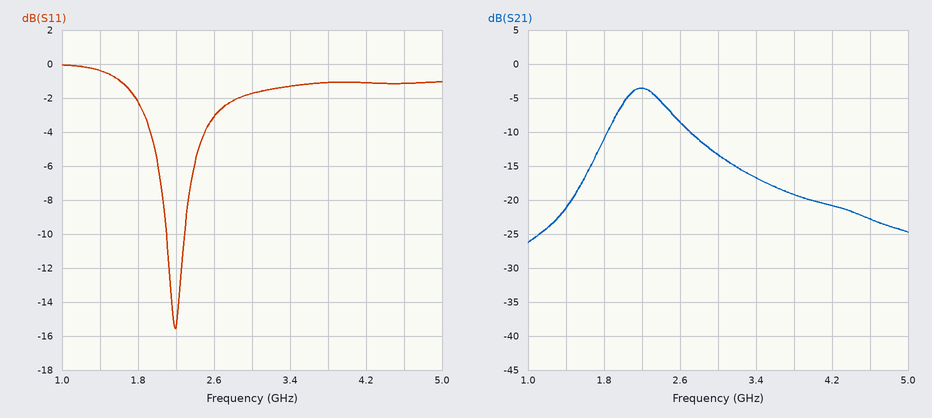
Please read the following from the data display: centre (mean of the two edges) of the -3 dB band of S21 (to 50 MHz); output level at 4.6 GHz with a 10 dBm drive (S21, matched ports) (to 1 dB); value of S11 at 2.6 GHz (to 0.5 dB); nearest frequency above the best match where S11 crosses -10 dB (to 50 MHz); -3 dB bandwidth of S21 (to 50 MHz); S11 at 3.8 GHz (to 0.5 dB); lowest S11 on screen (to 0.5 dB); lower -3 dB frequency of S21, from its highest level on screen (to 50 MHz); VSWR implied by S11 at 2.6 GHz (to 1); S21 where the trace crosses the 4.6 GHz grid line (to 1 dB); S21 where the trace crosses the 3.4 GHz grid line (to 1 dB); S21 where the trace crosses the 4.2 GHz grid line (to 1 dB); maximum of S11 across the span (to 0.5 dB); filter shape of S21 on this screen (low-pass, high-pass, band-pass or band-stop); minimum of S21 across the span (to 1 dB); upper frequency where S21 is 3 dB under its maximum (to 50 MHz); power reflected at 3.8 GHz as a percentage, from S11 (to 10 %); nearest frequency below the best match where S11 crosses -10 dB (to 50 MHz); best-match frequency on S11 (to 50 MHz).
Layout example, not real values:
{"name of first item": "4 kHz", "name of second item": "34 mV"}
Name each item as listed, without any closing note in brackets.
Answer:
{"centre (mean of the two edges) of the -3 dB band of S21": "2.20 GHz", "output level at 4.6 GHz with a 10 dBm drive (S21, matched ports)": "-13 dBm", "value of S11 at 2.6 GHz": "-3.0 dB", "nearest frequency above the best match where S11 crosses -10 dB": "2.30 GHz", "-3 dB bandwidth of S21": "500 MHz", "S11 at 3.8 GHz": "-1.0 dB", "lowest S11 on screen": "-15.5 dB", "lower -3 dB frequency of S21, from its highest level on screen": "1.95 GHz", "VSWR implied by S11 at 2.6 GHz": "6", "S21 where the trace crosses the 4.6 GHz grid line": "-23 dB", "S21 where the trace crosses the 3.4 GHz grid line": "-17 dB", "S21 where the trace crosses the 4.2 GHz grid line": "-21 dB", "maximum of S11 across the span": "0.0 dB", "filter shape of S21 on this screen": "band-pass", "minimum of S21 across the span": "-26 dB", "upper frequency where S21 is 3 dB under its maximum": "2.45 GHz", "power reflected at 3.8 GHz as a percentage, from S11": "80 %", "nearest frequency below the best match where S11 crosses -10 dB": "2.10 GHz", "best-match frequency on S11": "2.20 GHz"}
